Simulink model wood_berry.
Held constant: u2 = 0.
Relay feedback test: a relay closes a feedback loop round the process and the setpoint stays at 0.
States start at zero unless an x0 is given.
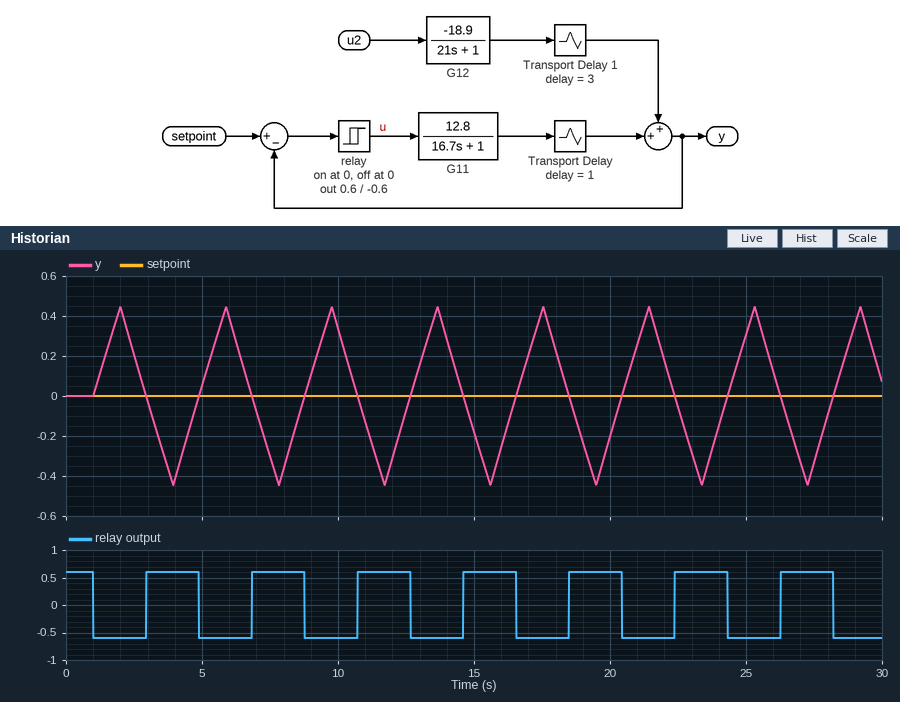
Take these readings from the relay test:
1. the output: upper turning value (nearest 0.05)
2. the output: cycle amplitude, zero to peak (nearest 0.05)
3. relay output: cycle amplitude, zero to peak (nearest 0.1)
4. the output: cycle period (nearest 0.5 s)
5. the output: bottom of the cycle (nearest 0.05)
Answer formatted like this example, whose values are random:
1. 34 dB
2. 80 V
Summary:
1. 0.45
2. 0.45
3. 0.6
4. 4.0 s
5. -0.45
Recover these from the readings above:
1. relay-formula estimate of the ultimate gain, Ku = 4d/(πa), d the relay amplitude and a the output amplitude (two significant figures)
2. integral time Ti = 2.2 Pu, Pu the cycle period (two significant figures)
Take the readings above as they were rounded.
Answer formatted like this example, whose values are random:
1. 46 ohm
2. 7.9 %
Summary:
1. 1.7
2. 8.8 s
